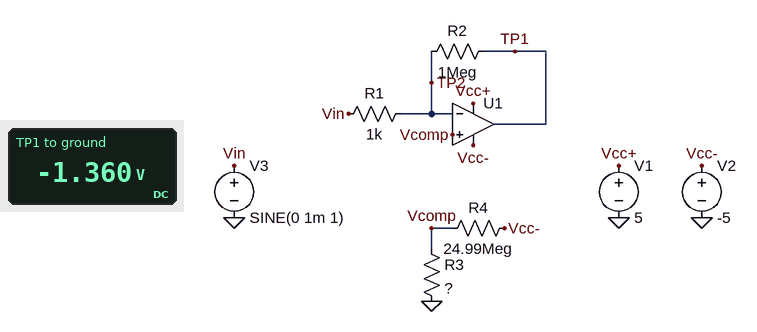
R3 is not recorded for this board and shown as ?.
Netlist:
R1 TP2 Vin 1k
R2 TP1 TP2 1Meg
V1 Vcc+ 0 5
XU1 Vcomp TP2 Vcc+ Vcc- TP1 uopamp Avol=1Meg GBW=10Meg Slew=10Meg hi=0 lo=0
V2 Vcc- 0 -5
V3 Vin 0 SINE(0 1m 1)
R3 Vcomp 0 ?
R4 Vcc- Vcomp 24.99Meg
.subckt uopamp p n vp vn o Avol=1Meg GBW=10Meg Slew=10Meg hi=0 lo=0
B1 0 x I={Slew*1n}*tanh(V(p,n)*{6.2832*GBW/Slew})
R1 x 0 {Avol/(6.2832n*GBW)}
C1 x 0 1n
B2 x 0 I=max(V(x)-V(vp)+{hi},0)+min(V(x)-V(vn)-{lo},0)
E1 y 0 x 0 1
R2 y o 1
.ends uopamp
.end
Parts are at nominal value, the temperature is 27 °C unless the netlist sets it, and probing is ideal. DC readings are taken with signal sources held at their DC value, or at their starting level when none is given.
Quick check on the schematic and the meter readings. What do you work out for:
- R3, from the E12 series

6.8 kΩ
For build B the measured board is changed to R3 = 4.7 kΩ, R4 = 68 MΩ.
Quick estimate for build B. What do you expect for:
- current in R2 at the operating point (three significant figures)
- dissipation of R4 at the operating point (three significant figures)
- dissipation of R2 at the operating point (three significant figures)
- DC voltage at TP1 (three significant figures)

345 nA
368 nW
119 nW
-346 mV
